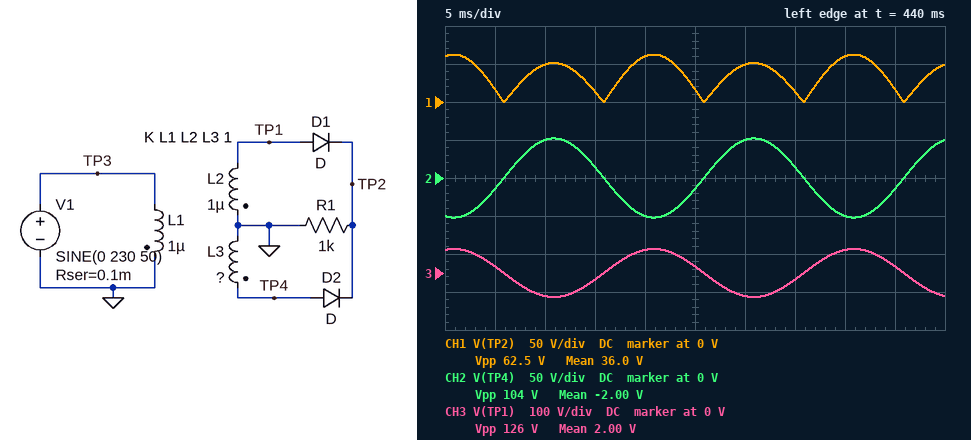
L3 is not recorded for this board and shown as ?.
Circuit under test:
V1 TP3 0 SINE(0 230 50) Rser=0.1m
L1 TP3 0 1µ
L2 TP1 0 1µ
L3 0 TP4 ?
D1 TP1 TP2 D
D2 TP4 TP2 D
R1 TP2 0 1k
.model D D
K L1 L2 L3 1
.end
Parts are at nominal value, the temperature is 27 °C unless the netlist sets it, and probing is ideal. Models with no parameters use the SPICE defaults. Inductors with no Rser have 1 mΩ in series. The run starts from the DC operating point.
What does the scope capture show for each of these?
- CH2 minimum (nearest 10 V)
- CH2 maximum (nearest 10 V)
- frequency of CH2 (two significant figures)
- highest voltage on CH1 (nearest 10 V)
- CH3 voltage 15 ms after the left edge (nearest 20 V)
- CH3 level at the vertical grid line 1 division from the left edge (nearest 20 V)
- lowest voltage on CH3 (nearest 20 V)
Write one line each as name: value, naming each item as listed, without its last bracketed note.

CH2 minimum: -50 V
CH2 maximum: 50 V
frequency of CH2: 50 Hz
highest voltage on CH1: 60 V
CH3 voltage 15 ms after the left edge: -20 V
CH3 level at the vertical grid line 1 division from the left edge: 20 V
lowest voltage on CH3: -60 V
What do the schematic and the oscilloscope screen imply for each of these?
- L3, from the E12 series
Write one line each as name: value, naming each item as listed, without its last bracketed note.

L3, from the E12 series: 680 nH
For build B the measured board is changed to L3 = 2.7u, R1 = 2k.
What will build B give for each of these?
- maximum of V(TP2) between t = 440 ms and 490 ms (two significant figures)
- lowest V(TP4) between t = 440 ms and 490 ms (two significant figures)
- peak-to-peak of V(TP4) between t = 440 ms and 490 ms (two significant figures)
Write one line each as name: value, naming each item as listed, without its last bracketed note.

maximum of V(TP2) between t = 440 ms and 490 ms: 100 V
lowest V(TP4) between t = 440 ms and 490 ms: -100 V
peak-to-peak of V(TP4) between t = 440 ms and 490 ms: 210 V
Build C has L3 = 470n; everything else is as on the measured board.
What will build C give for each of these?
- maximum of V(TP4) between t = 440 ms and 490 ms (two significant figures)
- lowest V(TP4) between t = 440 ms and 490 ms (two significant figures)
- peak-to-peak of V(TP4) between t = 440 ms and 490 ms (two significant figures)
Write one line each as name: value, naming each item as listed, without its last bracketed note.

maximum of V(TP4) between t = 440 ms and 490 ms: 43 V
lowest V(TP4) between t = 440 ms and 490 ms: -43 V
peak-to-peak of V(TP4) between t = 440 ms and 490 ms: 87 V
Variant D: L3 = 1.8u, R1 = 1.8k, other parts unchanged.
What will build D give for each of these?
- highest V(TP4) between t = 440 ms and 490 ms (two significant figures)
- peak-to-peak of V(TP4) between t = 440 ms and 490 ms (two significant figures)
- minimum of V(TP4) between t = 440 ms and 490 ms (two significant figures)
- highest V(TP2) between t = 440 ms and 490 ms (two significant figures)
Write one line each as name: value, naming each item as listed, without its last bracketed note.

highest V(TP4) between t = 440 ms and 490 ms: 85 V
peak-to-peak of V(TP4) between t = 440 ms and 490 ms: 170 V
minimum of V(TP4) between t = 440 ms and 490 ms: -85 V
highest V(TP2) between t = 440 ms and 490 ms: 84 V
